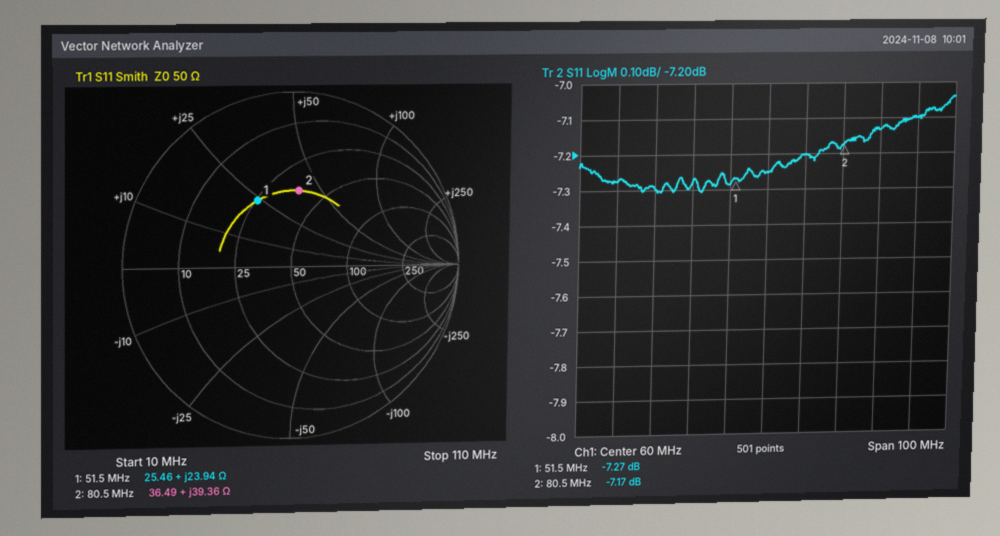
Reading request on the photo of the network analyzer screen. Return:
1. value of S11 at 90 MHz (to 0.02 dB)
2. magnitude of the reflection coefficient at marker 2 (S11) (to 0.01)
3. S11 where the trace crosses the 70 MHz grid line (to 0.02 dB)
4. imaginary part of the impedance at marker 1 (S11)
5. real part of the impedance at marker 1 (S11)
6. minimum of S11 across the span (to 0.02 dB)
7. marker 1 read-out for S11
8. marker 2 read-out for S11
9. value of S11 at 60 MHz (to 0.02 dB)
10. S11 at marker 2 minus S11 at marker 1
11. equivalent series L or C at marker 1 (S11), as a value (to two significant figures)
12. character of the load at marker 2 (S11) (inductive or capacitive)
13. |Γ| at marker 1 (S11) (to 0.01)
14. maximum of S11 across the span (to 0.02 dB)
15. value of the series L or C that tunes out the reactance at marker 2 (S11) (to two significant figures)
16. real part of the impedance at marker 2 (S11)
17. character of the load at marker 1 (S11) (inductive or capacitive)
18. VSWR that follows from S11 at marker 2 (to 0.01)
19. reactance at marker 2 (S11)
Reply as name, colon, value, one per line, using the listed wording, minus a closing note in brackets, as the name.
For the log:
value of S11 at 90 MHz: -7.14 dB
magnitude of the reflection coefficient at marker 2 (S11): 0.44
S11 where the trace crosses the 70 MHz grid line: -7.20 dB
imaginary part of the impedance at marker 1: +23.94 Ω
real part of the impedance at marker 1: 25.46 Ω
minimum of S11 across the span: -7.30 dB
marker 1 read-out for S11: -7.27 dB
marker 2 read-out for S11: -7.17 dB
value of S11 at 60 MHz: -7.26 dB
S11 at marker 2 minus S11 at marker 1: 0.10 dB
equivalent series L or C at marker 1 (S11), as a value: 74 nH
character of the load at marker 2 (S11): inductive
|Γ| at marker 1 (S11): 0.43
maximum of S11 across the span: -7.04 dB
value of the series L or C that tunes out the reactance at marker 2 (S11): 50 pF
real part of the impedance at marker 2: 36.49 Ω
character of the load at marker 1 (S11): inductive
VSWR that follows from S11 at marker 2: 2.56
reactance at marker 2: +39.36 Ω
